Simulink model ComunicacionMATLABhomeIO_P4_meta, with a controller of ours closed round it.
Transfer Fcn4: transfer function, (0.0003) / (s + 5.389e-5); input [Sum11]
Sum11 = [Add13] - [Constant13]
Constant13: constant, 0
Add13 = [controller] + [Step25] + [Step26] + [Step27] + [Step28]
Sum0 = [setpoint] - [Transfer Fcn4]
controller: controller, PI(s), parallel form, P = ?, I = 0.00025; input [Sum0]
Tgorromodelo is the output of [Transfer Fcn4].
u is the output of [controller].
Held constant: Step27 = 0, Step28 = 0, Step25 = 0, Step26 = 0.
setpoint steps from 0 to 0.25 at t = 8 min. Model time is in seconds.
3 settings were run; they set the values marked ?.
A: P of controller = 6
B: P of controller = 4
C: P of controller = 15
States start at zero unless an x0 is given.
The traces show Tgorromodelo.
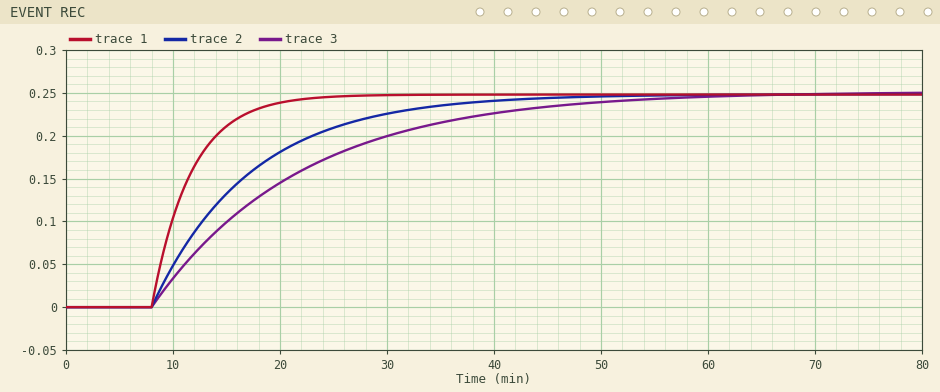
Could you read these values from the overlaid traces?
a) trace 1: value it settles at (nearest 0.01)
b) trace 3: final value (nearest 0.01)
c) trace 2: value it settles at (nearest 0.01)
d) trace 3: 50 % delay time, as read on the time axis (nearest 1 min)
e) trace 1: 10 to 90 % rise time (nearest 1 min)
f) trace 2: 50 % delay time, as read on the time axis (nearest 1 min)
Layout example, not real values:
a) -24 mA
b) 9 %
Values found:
a) 0.25
b) 0.25
c) 0.25
d) 18 min
e) 8 min
f) 14 min
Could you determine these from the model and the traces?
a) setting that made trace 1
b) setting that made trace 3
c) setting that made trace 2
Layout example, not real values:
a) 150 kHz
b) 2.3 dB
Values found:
a) C
b) B
c) A
